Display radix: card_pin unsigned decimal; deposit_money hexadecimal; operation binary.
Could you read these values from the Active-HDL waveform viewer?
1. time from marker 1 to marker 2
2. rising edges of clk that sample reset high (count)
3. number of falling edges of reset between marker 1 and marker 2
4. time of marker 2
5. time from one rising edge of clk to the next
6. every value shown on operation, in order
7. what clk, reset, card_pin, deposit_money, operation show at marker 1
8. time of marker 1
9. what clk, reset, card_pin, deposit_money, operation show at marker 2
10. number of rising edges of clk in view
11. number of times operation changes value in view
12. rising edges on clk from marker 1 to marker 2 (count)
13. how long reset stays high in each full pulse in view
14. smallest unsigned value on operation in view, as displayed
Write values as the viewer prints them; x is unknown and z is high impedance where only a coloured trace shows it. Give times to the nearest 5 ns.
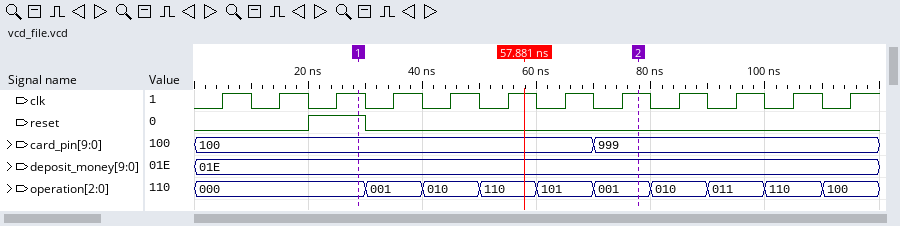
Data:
50 ns
1
1
80 ns
10 ns
000, 001, 010, 110, 101, 001, 010, 011, 110, 100
clk=1, reset=1, card_pin=100, deposit_money=01E, operation=000
30 ns
clk=1, reset=0, card_pin=999, deposit_money=01E, operation=001
12
9
5
10 ns
000
